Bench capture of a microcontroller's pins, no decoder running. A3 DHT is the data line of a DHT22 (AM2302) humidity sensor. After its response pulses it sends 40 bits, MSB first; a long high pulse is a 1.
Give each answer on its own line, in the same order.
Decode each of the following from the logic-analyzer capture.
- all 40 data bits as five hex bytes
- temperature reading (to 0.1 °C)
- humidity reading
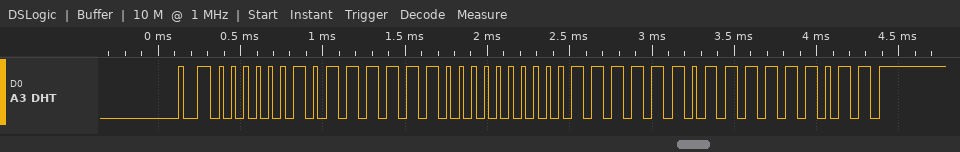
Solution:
02 FC 00 FD FB
25.3 °C
76.4 %
